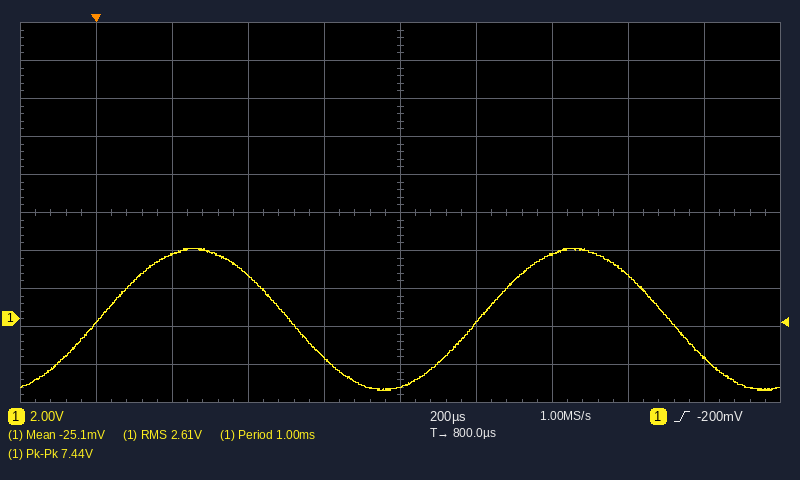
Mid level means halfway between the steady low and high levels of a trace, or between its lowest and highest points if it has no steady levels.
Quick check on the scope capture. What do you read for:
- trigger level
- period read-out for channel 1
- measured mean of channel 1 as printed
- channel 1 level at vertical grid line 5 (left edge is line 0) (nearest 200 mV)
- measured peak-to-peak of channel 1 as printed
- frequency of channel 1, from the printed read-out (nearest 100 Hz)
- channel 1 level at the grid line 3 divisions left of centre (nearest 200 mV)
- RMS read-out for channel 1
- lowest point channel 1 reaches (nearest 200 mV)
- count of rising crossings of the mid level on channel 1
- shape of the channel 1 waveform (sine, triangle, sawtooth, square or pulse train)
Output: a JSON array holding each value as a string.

["-200 mV", "1.00 ms", "-25.1 mV", "-3.6 V", "7.44 V", "1.0 kHz", "3.4 V", "2.61 V", "-3.8 V", "2", "sine"]
